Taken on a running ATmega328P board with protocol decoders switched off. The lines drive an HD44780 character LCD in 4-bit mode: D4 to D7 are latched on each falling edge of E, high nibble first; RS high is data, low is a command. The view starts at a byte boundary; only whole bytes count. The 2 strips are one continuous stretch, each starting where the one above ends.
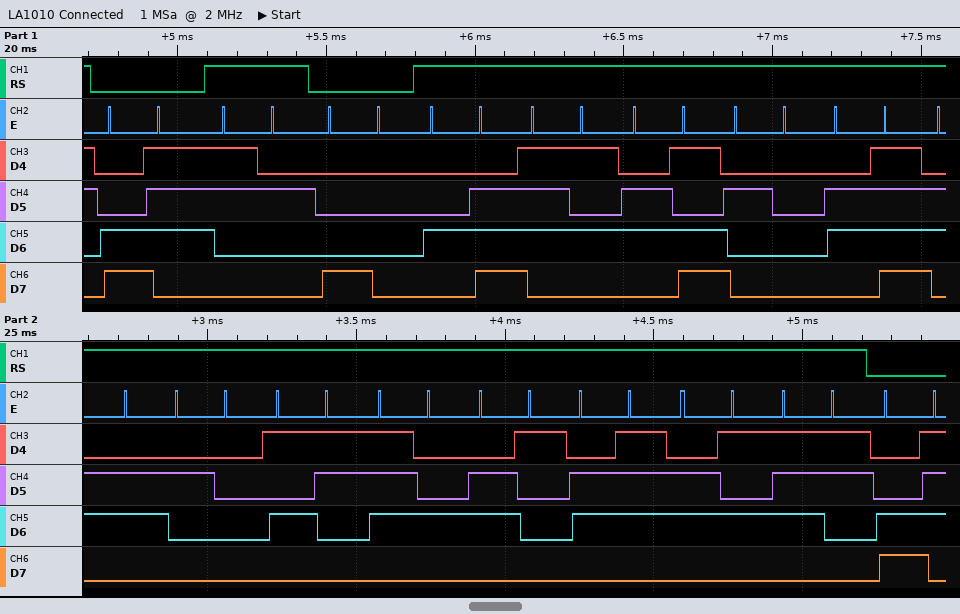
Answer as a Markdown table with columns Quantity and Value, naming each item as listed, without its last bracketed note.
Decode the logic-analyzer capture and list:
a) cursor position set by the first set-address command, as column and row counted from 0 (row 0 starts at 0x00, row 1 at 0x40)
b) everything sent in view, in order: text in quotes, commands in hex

| Quantity | Value |
|---|---|
| cursor position set by the first set-address command, as column and row counted from 0 | column 7, row 1 |
| everything sent in view, in order: text in quotes, commands in hex | 0xC7 "2" 0x80 "Num of Stages" 0xC7 |
